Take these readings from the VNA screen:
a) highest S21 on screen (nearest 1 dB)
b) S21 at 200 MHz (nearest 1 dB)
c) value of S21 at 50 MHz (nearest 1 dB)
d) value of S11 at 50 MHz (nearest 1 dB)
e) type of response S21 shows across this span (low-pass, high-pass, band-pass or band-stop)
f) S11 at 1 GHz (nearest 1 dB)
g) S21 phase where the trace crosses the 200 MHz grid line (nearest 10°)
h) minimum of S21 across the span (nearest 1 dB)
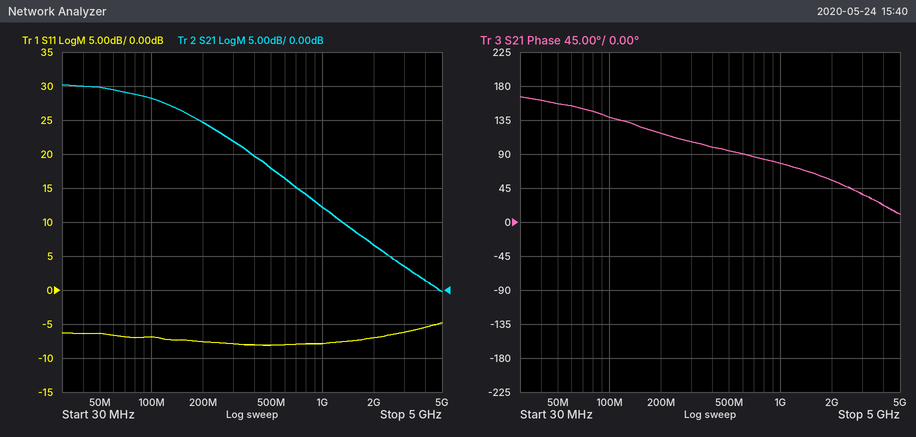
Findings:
30 dB
25 dB
30 dB
-6 dB
low-pass
-8 dB
120°
0 dB
